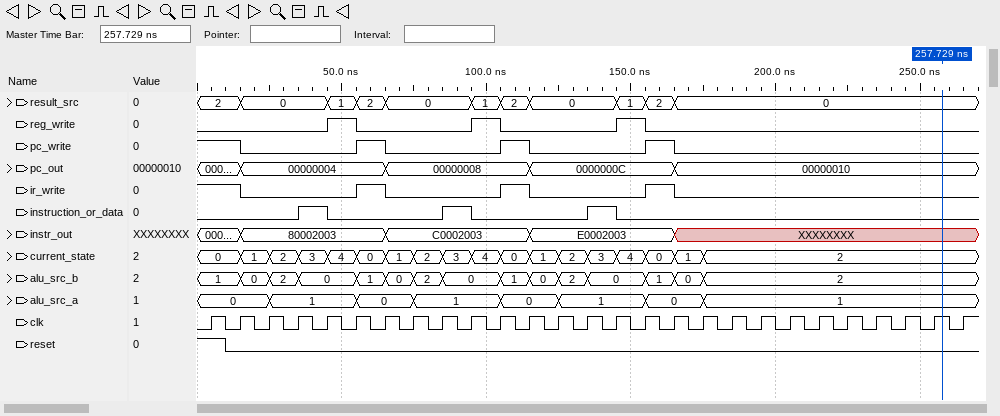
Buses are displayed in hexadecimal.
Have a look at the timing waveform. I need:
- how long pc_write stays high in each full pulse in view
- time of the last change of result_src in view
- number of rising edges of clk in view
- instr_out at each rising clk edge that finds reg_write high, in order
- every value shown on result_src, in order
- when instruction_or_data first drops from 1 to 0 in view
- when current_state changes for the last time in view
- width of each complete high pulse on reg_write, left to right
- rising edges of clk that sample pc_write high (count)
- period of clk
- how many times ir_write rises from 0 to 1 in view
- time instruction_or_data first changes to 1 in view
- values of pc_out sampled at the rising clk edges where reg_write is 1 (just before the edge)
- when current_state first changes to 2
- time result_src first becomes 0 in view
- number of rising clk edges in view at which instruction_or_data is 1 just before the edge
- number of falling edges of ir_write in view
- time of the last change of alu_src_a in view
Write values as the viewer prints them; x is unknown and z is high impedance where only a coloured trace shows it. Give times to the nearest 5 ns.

10 ns, 10 ns, 10 ns
165 ns
27
80002003, C0002003, E0002003
2, 0, 1, 2, 0, 1, 2, 0, 1, 2, 0
45 ns
175 ns
10 ns, 10 ns, 10 ns
5
10 ns
3
35 ns
00000004, 00000008, 0000000C
25 ns
15 ns
3
4
175 ns
